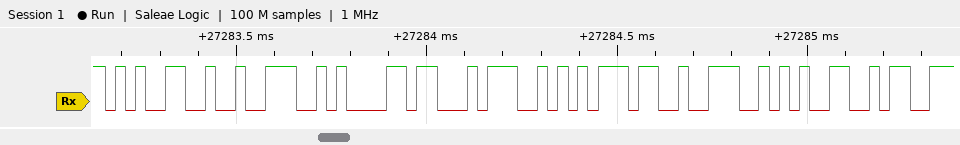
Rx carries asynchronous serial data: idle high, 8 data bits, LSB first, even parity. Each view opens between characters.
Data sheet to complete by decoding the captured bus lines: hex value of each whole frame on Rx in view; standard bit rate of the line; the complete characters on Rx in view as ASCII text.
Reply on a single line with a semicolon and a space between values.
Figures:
65, 72, 61, 74, 75, 72, 65; 38400 baud; "erature"
